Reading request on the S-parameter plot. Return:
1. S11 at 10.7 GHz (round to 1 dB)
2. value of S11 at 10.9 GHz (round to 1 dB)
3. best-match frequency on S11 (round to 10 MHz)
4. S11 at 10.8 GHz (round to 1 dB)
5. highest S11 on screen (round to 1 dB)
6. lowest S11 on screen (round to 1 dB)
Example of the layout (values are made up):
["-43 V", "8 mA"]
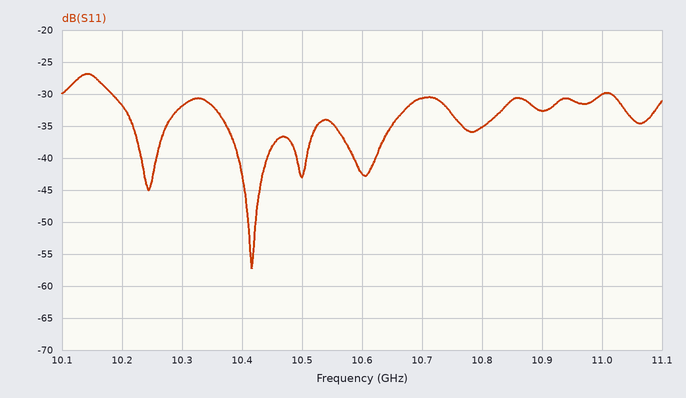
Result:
["-31 dB", "-33 dB", "10.42 GHz", "-35 dB", "-27 dB", "-57 dB"]
